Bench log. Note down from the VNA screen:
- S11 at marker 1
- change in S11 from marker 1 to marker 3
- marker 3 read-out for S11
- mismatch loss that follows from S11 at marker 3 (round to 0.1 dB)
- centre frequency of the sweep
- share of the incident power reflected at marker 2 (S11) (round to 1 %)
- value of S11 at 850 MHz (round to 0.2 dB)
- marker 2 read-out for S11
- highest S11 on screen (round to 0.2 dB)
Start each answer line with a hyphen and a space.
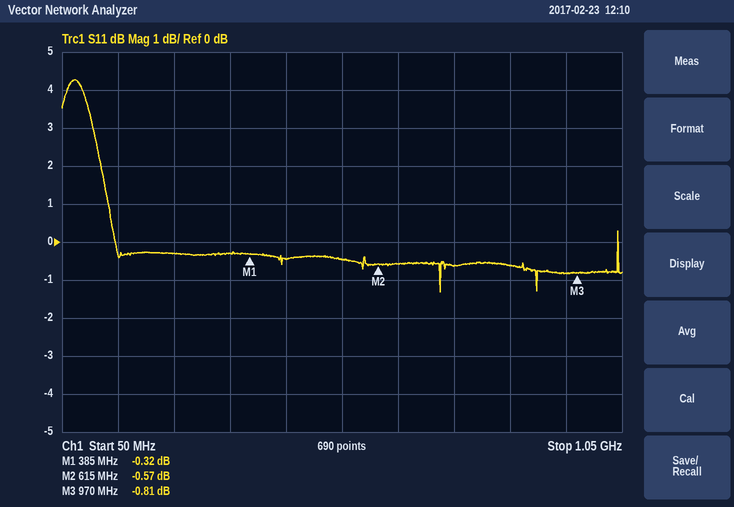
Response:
- -0.32 dB
- -0.49 dB
- -0.81 dB
- 7.7 dB
- 550 MHz
- 88 %
- -0.6 dB
- -0.57 dB
- 4.2 dB
